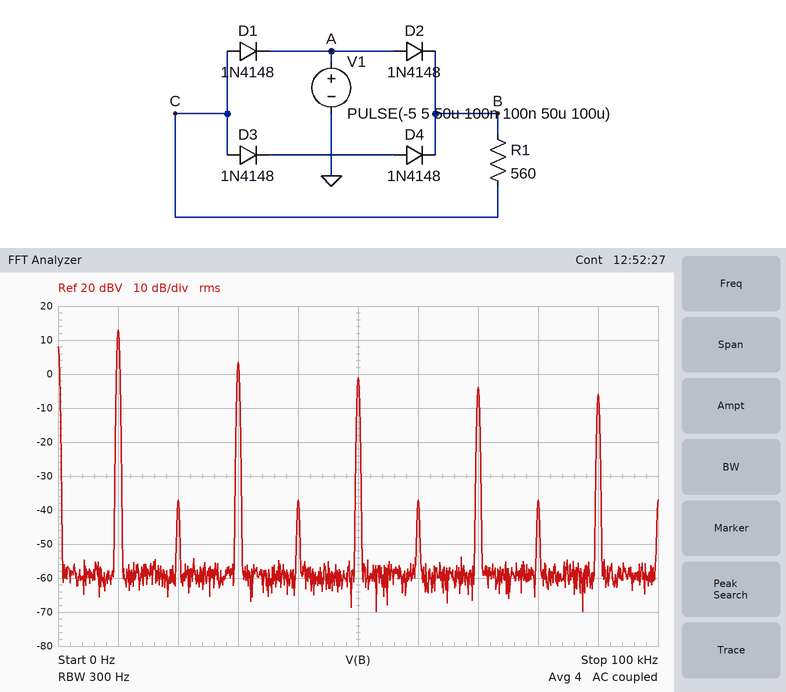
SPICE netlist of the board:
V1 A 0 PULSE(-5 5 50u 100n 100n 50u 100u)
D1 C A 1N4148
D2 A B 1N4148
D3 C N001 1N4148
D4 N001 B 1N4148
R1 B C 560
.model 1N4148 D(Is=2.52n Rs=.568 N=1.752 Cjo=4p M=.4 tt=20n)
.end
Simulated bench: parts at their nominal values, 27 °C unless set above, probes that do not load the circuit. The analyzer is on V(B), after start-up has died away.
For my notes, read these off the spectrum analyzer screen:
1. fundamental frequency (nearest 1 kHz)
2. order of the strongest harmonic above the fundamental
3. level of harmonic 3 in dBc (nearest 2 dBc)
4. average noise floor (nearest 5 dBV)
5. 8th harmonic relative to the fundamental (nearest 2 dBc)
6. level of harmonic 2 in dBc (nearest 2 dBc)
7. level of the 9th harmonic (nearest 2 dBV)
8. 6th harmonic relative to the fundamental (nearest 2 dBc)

10 kHz
3
-10 dBc
-60 dBV
-50 dBc
-50 dBc
-6 dBV
-50 dBc
